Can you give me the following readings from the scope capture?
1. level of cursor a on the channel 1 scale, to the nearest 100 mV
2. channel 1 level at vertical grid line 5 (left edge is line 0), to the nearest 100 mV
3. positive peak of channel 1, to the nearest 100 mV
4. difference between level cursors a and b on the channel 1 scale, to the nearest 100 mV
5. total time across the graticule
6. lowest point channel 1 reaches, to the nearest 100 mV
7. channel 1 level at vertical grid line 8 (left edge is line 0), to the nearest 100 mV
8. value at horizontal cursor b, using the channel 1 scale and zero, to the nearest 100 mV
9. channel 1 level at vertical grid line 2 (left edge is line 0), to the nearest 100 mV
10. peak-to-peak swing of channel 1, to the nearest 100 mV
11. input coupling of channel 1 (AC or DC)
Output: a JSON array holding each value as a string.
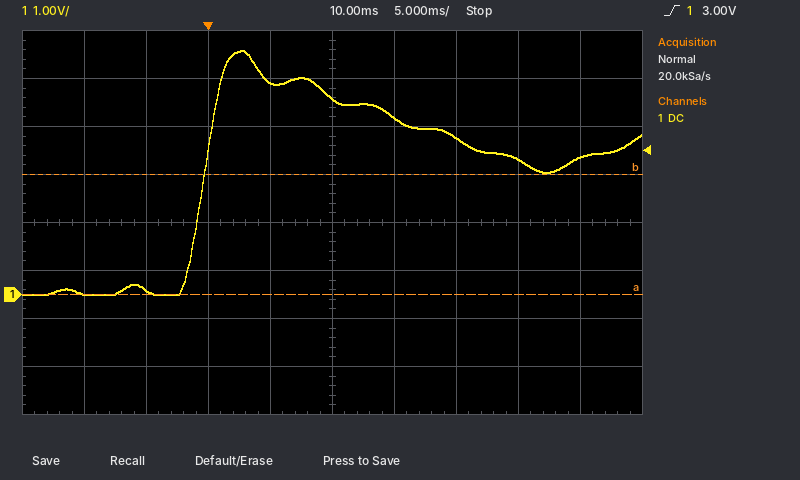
["0.0 V", "4.1 V", "5.1 V", "2.5 V", "50 ms", "0.0 V", "2.8 V", "2.5 V", "100 mV", "5.1 V", "DC"]
